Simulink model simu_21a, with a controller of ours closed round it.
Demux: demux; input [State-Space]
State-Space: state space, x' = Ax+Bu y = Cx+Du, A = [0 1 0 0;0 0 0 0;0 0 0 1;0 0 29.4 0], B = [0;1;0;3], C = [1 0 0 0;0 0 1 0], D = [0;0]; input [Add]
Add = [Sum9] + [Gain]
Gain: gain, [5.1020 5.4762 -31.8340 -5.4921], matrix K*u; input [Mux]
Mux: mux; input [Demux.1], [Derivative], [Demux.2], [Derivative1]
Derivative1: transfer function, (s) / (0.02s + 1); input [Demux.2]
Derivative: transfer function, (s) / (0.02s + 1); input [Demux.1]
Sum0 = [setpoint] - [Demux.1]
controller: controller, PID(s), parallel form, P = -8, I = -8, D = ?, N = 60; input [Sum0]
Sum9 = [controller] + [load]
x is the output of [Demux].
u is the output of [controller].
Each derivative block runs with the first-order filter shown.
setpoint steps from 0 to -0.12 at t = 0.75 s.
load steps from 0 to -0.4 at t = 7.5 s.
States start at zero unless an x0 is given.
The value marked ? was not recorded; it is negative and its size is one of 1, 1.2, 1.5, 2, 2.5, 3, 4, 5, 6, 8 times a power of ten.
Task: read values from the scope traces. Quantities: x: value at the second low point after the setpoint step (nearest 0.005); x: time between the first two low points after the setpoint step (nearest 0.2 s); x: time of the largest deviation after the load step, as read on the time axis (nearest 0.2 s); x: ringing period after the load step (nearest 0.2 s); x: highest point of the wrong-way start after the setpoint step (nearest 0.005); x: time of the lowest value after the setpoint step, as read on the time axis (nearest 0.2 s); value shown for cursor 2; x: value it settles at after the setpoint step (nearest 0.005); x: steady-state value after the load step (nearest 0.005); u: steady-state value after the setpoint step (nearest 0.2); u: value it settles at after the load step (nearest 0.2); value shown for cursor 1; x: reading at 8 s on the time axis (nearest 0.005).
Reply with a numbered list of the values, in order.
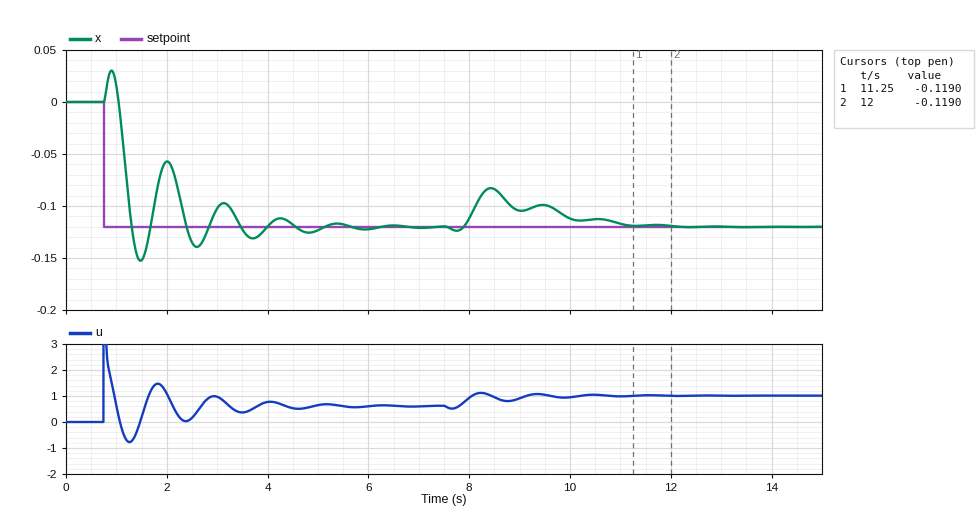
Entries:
1. -0.140
2. 1.2 s
3. 8.4 s
4. 1.0 s
5. 0.030
6. 1.4 s
7. -0.1190
8. -0.120
9. -0.120
10. 0.6
11. 1.0
12. -0.1190
13. -0.110
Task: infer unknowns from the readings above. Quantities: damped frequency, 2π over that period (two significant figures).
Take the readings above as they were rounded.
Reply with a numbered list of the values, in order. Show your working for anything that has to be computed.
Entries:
1. 2π / 1.2 = 5.2 rad/s
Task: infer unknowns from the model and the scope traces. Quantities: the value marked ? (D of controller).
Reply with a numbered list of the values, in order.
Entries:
1. -3
